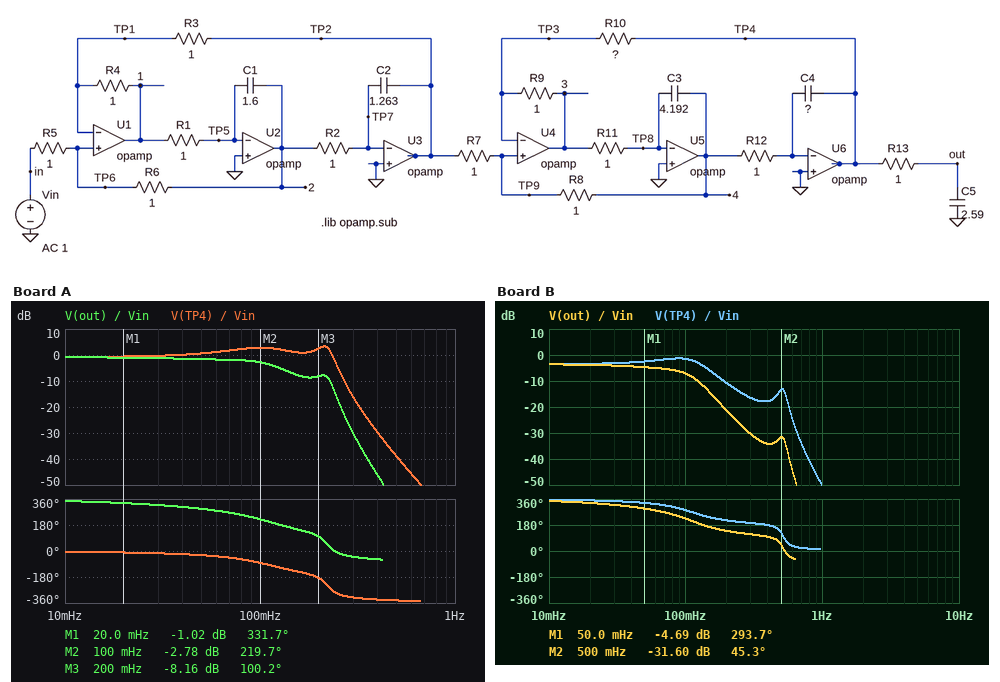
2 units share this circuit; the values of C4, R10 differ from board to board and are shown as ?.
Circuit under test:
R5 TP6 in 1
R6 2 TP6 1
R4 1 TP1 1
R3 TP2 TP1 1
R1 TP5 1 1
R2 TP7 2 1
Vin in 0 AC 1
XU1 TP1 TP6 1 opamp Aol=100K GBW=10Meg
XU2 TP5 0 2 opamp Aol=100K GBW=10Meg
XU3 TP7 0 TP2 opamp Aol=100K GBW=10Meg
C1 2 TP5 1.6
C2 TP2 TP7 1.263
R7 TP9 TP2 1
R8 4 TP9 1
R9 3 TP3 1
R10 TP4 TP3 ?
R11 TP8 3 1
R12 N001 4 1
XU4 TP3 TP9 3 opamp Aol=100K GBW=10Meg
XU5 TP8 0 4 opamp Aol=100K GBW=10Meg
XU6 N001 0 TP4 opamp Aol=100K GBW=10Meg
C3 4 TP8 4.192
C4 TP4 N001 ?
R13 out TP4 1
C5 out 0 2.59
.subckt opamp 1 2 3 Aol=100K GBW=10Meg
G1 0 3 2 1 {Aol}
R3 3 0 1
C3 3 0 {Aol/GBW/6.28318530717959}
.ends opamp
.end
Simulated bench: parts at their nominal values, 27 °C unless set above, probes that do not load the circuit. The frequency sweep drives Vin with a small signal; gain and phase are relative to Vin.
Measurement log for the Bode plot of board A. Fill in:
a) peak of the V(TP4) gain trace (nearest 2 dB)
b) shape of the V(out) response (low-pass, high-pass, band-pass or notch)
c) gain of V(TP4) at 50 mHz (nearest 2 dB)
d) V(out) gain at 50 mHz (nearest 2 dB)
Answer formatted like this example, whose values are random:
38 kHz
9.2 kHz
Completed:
4 dB
low-pass
0 dB
-2 dB
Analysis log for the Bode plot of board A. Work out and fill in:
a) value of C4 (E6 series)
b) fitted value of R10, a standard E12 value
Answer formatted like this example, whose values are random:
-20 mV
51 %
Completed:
150 mF
0.82 Ω
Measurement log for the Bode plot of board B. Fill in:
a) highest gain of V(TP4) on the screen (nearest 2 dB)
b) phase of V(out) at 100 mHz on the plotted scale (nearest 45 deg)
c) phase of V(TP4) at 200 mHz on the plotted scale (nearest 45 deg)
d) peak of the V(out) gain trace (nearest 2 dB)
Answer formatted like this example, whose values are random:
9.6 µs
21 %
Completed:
-2 dB
225 deg
225 deg
-4 dB
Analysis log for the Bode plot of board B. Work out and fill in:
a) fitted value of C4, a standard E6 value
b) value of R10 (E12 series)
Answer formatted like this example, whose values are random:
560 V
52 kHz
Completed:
68 mF
0.33 Ω
